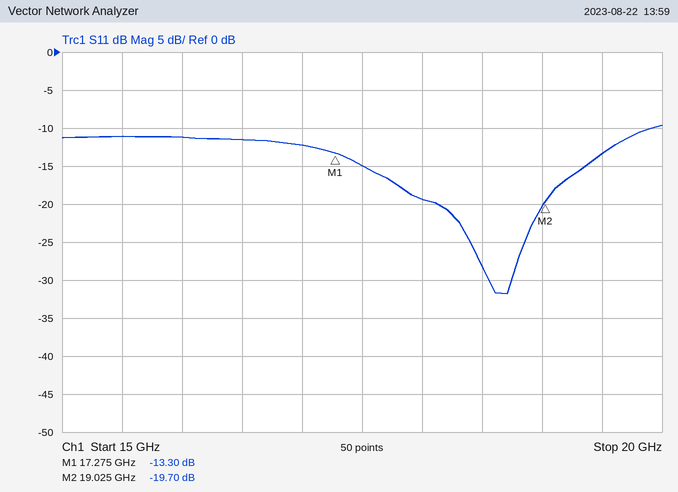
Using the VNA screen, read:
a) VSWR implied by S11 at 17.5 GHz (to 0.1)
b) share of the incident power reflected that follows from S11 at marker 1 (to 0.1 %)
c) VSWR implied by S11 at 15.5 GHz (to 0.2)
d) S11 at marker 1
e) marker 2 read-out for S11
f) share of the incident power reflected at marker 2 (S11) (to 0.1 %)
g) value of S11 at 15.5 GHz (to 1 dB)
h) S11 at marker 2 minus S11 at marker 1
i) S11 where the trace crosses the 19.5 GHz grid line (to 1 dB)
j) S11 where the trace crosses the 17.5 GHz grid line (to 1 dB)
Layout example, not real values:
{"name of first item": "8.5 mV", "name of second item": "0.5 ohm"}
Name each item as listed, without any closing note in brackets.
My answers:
{"VSWR implied by S11 at 17.5 GHz": "1.4", "share of the incident power reflected that follows from S11 at marker 1": "4.7 %", "VSWR implied by S11 at 15.5 GHz": "1.8", "S11 at marker 1": "-13.30 dB", "marker 2 read-out for S11": "-19.70 dB", "share of the incident power reflected at marker 2 (S11)": "1.1 %", "value of S11 at 15.5 GHz": "-11 dB", "S11 at marker 2 minus S11 at marker 1": "-6.40 dB", "S11 where the trace crosses the 19.5 GHz grid line": "-13 dB", "S11 where the trace crosses the 17.5 GHz grid line": "-15 dB"}
